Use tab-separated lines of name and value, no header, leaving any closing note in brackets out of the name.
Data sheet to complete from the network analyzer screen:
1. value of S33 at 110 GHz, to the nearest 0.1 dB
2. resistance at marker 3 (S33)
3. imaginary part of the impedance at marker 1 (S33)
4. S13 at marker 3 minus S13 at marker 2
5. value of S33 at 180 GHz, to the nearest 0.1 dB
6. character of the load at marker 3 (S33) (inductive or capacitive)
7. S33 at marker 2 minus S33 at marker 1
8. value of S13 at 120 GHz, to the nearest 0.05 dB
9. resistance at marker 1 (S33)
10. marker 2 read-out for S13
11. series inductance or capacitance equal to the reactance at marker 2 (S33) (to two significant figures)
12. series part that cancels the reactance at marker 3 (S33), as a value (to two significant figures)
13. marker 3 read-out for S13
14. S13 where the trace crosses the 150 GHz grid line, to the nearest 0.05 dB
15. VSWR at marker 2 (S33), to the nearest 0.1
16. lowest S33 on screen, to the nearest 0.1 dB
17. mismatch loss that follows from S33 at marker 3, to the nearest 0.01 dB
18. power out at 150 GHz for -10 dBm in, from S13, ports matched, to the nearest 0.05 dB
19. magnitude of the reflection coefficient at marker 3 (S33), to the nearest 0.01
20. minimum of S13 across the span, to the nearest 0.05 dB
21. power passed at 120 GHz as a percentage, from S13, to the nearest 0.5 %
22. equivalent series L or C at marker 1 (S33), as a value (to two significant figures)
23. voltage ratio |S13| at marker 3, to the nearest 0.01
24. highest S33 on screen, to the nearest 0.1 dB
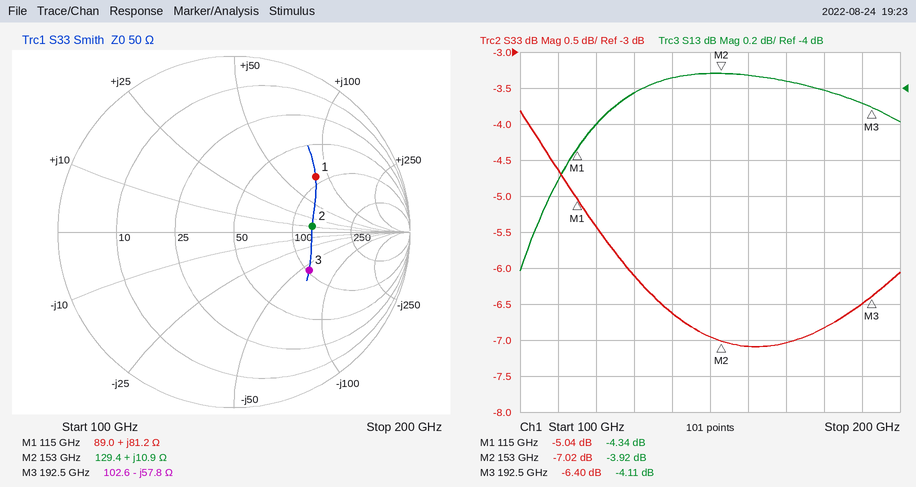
value of S33 at 110 GHz, to the nearest 0.1 dB	-4.6 dB
resistance at marker 3	102.6 Ω
imaginary part of the impedance at marker 1	+81.2 Ω
S13 at marker 3 minus S13 at marker 2	-0.19 dB
value of S33 at 180 GHz, to the nearest 0.1 dB	-6.8 dB
character of the load at marker 3 (S33)	capacitive
S33 at marker 2 minus S33 at marker 1	-1.98 dB
value of S13 at 120 GHz, to the nearest 0.05 dB	-4.20 dB
resistance at marker 1	89.0 Ω
marker 2 read-out for S13	-3.92 dB
series inductance or capacitance equal to the reactance at marker 2 (S33)	11 pH
series part that cancels the reactance at marker 3 (S33), as a value	48 pH
marker 3 read-out for S13	-4.11 dB
S13 where the trace crosses the 150 GHz grid line, to the nearest 0.05 dB	-3.90 dB
VSWR at marker 2 (S33), to the nearest 0.1	2.6
lowest S33 on screen, to the nearest 0.1 dB	-7.1 dB
mismatch loss that follows from S33 at marker 3, to the nearest 0.01 dB	1.13 dB
power out at 150 GHz for -10 dBm in, from S13, ports matched, to the nearest 0.05 dB	-13.90 dBm
magnitude of the reflection coefficient at marker 3 (S33), to the nearest 0.01	0.48
minimum of S13 across the span, to the nearest 0.05 dB	-5.00 dB
power passed at 120 GHz as a percentage, from S13, to the nearest 0.5 %	38.0 %
equivalent series L or C at marker 1 (S33), as a value	110 pH
voltage ratio |S13| at marker 3, to the nearest 0.01	0.62
highest S33 on screen, to the nearest 0.1 dB	-3.8 dB
